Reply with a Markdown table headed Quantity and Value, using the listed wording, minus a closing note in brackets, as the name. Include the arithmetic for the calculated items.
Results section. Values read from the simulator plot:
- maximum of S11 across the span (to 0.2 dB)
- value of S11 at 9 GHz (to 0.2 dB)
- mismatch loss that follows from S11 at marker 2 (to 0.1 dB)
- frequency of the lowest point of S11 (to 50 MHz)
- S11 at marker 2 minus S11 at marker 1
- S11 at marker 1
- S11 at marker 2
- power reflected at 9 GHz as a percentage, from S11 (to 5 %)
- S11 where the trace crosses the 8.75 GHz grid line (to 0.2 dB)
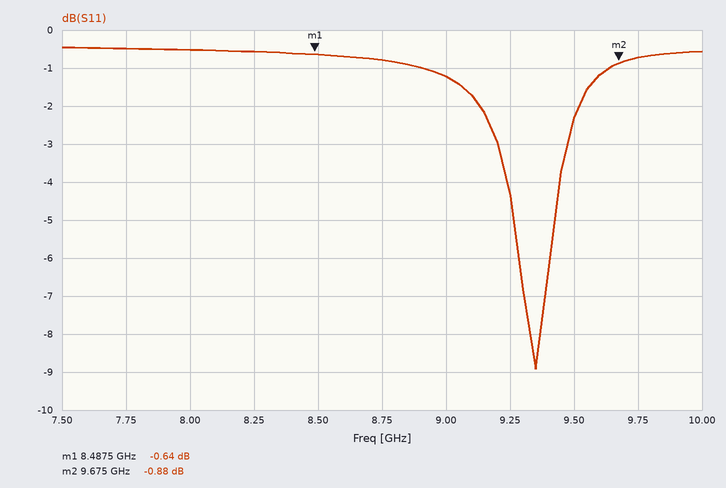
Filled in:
| Quantity | Value |
|---|---|
| maximum of S11 across the span | -0.4 dB |
| value of S11 at 9 GHz | -1.2 dB |
| mismatch loss that follows from S11 at marker 2 | −10 log10(1 − 10^(-0.88/10)) ≈ 7.4 dB |
| frequency of the lowest point of S11 | 9.35 GHz |
| S11 at marker 2 minus S11 at marker 1 | -0.88 − (-0.64) = -0.24 dB |
| S11 at marker 1 | -0.64 dB |
| S11 at marker 2 | -0.88 dB |
| power reflected at 9 GHz as a percentage, from S11 | 10^(-1.2/10) ≈ 75.9 %, so 75 % to the nearest 5 % |
| S11 where the trace crosses the 8.75 GHz grid line | -0.8 dB |
